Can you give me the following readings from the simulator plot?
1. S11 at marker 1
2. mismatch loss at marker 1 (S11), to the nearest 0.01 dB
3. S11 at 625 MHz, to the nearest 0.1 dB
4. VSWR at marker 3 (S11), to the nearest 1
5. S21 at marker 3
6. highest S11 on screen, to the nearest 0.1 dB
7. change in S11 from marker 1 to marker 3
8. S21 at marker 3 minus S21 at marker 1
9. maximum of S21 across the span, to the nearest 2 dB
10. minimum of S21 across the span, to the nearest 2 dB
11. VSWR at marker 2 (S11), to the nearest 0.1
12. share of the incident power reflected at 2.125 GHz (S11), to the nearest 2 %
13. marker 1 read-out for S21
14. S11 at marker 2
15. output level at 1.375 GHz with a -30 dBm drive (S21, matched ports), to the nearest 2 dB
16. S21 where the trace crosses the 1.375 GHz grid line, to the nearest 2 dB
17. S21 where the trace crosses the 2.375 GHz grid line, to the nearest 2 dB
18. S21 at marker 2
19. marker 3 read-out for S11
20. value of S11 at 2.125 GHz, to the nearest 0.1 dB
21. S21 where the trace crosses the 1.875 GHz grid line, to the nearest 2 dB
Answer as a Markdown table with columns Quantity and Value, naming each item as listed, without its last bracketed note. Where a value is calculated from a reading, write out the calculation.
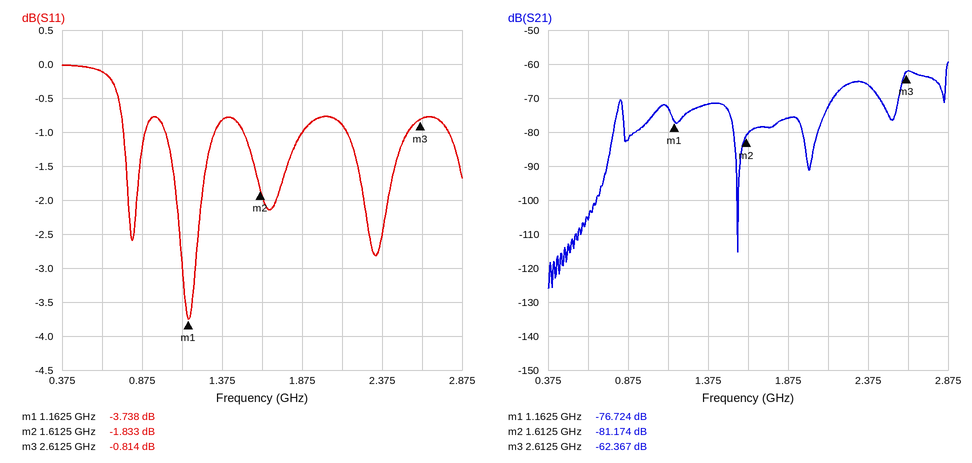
| Quantity | Value |
|---|---|
| S11 at marker 1 | -3.738 dB |
| mismatch loss at marker 1 (S11), to the nearest 0.01 dB | −10 log10(1 − 10^(-3.738/10)) ≈ 2.39 dB |
| S11 at 625 MHz, to the nearest 0.1 dB | -0.1 dB |
| VSWR at marker 3 (S11), to the nearest 1 | (1 + 0.9105)/(1 − 0.9105) ≈ 21 |
| S21 at marker 3 | -62.367 dB |
| highest S11 on screen, to the nearest 0.1 dB | 0.0 dB |
| change in S11 from marker 1 to marker 3 | -0.814 − (-3.738) = 2.924 dB |
| S21 at marker 3 minus S21 at marker 1 | -62.367 − (-76.724) = 14.357 dB |
| maximum of S21 across the span, to the nearest 2 dB | -60 dB |
| minimum of S21 across the span, to the nearest 2 dB | -126 dB |
| VSWR at marker 2 (S11), to the nearest 0.1 | (1 + 0.8097)/(1 − 0.8097) ≈ 9.5 |
| share of the incident power reflected at 2.125 GHz (S11), to the nearest 2 % | 10^(-0.9/10) ≈ 81.3 %, so 82 % to the nearest 2 % |
| marker 1 read-out for S21 | -76.724 dB |
| S11 at marker 2 | -1.833 dB |
| output level at 1.375 GHz with a -30 dBm drive (S21, matched ports), to the nearest 2 dB | -30 dBm + (-72 dB) = -102 dBm |
| S21 where the trace crosses the 1.375 GHz grid line, to the nearest 2 dB | -72 dB |
| S21 where the trace crosses the 2.375 GHz grid line, to the nearest 2 dB | -66 dB |
| S21 at marker 2 | -81.174 dB |
| marker 3 read-out for S11 | -0.814 dB |
| value of S11 at 2.125 GHz, to the nearest 0.1 dB | -0.9 dB |
| S21 where the trace crosses the 1.875 GHz grid line, to the nearest 2 dB | -76 dB |
